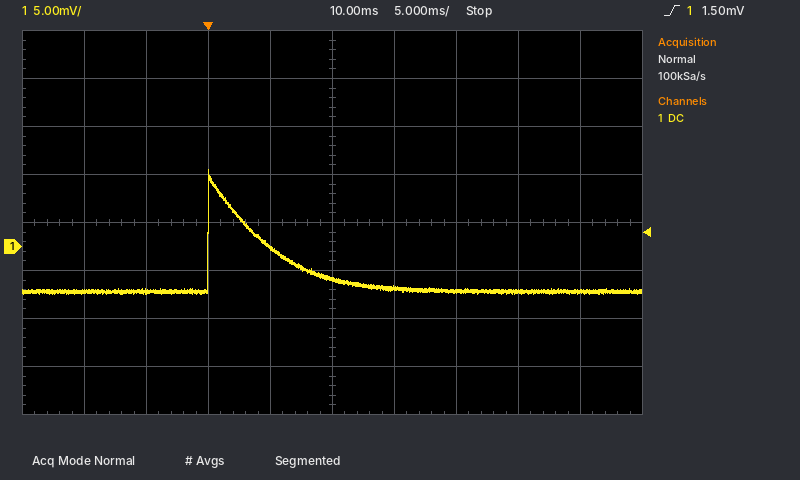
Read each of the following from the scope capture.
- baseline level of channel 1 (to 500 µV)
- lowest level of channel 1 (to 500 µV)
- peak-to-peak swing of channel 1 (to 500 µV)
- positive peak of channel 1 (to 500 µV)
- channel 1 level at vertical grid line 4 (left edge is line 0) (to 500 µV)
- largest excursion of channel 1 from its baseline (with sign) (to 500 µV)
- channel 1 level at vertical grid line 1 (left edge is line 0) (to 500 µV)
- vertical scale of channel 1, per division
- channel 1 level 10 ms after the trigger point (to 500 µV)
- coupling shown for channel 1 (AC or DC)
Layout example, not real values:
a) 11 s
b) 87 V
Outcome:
a) -4.5 mV
b) -5.0 mV
c) 13.0 mV
d) 8.0 mV
e) 0.0 mV
f) +12.5 mV
g) -4.5 mV
h) 5 mV
i) -3.5 mV
j) DC
